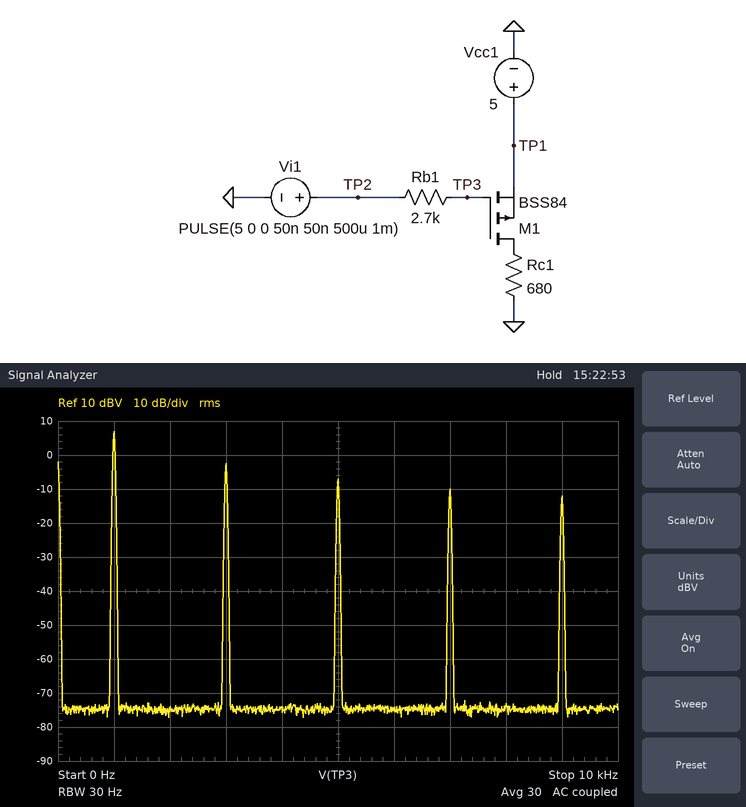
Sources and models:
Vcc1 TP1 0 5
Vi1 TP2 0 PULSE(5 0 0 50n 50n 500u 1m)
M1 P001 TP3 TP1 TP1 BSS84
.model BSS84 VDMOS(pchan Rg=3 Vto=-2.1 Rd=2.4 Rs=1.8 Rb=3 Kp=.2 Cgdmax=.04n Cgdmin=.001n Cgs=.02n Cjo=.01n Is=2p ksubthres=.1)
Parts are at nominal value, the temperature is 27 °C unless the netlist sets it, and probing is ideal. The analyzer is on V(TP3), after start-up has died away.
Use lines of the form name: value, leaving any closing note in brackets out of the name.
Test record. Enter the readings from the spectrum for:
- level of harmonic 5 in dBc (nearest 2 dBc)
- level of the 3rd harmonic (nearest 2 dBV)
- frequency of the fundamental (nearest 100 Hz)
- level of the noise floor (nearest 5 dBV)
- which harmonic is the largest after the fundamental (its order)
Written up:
level of harmonic 5 in dBc: -14 dBc
level of the 3rd harmonic: -2 dBV
frequency of the fundamental: 1.0 kHz
level of the noise floor: -75 dBV
which harmonic is the largest after the fundamental: 3
